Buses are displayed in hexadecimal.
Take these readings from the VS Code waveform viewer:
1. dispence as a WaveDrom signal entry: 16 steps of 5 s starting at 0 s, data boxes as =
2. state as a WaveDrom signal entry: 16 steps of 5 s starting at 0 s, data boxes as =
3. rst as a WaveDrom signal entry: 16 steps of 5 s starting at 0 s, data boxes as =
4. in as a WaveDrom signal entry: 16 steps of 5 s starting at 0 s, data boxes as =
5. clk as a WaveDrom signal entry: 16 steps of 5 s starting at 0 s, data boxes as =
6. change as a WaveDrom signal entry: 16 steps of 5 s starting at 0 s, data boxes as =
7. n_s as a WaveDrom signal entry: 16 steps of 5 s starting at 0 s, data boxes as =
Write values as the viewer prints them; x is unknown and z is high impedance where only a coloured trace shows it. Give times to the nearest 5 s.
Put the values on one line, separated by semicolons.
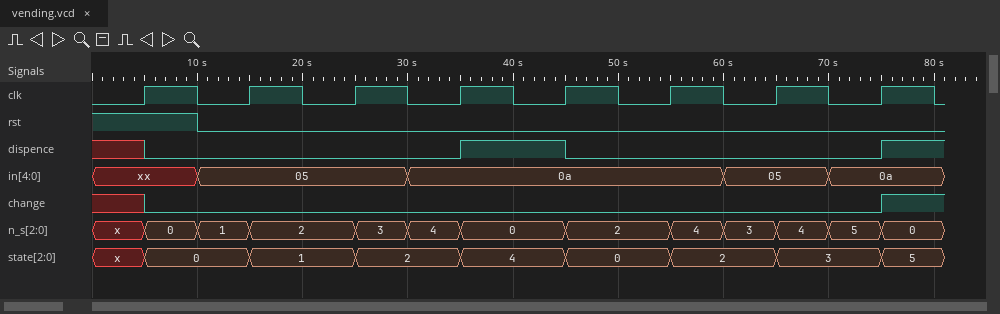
{name: 'dispence', wave: 'x0.....1.0.....1'}; {name: 'state', wave: 'x=.=.=.=.=.=.=.=', data: '0 1 2 4 0 2 3 5'}; {name: 'rst', wave: '1.0.............'}; {name: 'in', wave: 'x.=...=.....=.=.', data: '05 0a 05 0a'}; {name: 'clk', wave: '0101010101010101'}; {name: 'change', wave: 'x0.............1'}; {name: 'n_s', wave: 'x===.===.=.=====', data: '0 1 2 3 4 0 2 4 3 4 5 0'}
